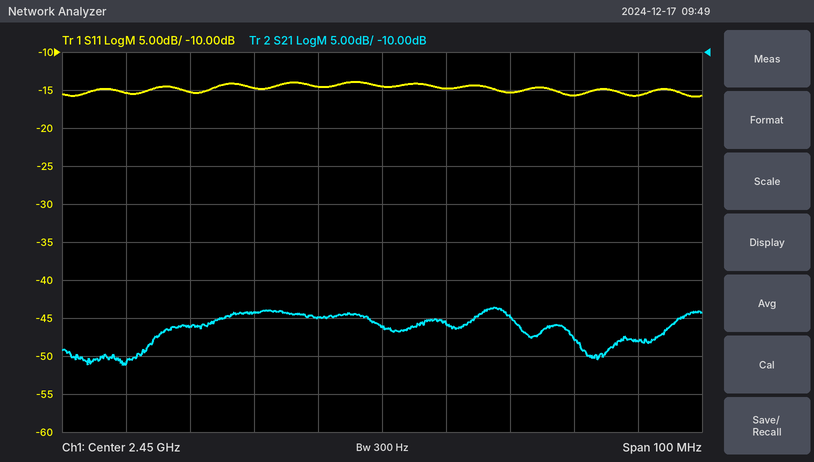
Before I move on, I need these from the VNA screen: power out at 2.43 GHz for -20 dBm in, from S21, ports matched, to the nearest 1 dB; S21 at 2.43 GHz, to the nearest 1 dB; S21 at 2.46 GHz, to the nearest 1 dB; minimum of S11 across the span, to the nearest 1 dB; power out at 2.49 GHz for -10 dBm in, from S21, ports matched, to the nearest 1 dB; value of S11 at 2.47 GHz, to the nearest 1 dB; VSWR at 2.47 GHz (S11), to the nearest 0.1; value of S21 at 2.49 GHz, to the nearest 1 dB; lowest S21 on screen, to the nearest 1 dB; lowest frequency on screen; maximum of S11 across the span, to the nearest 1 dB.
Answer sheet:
-64 dBm
-44 dB
-46 dB
-16 dB
-58 dBm
-15 dB
1.4
-48 dB
-51 dB
2.4 GHz
-14 dB
